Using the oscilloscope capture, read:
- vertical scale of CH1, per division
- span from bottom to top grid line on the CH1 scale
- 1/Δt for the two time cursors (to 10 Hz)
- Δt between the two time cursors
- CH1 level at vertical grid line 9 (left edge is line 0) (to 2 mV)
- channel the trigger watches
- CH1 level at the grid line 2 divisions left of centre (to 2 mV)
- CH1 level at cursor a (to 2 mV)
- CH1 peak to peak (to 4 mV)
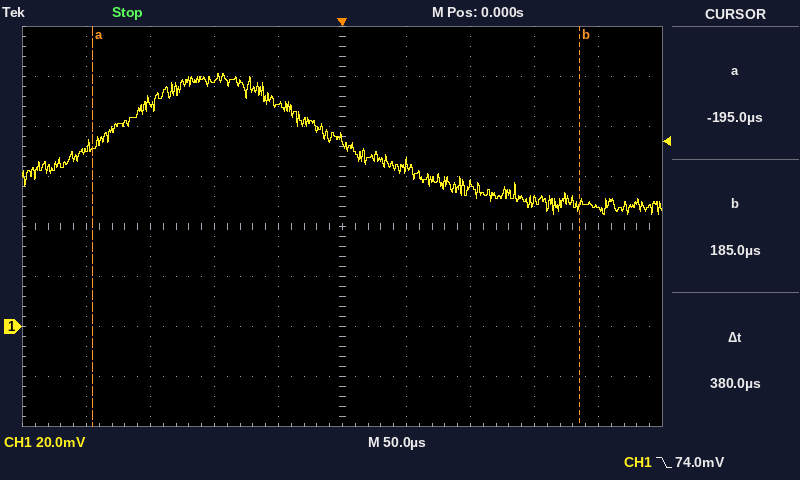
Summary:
20 mV
160 mV
2.63 kHz
380 µs
48 mV
CH1
98 mV
72 mV
56 mV
